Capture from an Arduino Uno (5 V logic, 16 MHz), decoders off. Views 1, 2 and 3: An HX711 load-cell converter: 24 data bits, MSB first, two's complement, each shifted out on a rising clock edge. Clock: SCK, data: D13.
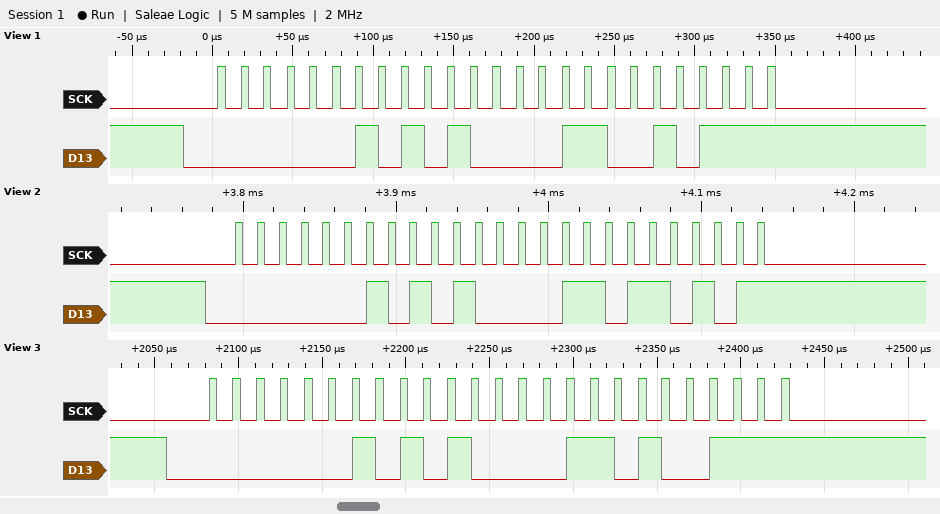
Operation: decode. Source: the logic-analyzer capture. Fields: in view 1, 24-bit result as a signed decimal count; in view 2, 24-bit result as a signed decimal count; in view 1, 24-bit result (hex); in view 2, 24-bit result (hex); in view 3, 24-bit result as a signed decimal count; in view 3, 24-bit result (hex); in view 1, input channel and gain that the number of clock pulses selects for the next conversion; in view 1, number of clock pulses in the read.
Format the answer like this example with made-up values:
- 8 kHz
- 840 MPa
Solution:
- 172439
- 172469
- 0x02A197
- 0x02A1B5
- 172455
- 0x02A1A7
- channel A, gain 128
- 25
